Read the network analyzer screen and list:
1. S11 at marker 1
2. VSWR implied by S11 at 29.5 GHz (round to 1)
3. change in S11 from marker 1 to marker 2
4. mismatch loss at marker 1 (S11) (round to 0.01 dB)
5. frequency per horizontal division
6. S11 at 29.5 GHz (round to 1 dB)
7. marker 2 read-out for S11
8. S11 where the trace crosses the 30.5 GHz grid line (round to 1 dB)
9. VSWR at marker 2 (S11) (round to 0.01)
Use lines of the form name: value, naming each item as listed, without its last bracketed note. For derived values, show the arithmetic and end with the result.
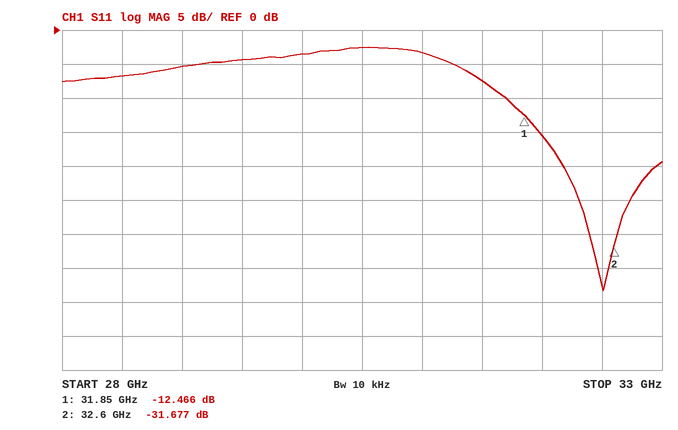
S11 at marker 1: -12.466 dB
VSWR implied by S11 at 29.5 GHz: |Γ| = 10^(-4/20) = 0.6310; VSWR = (1 + 0.6310)/(1 − 0.6310) ≈ 4
change in S11 from marker 1 to marker 2: -31.677 − (-12.466) = -19.211 dB
mismatch loss at marker 1 (S11): −10 log10(1 − 10^(-12.466/10)) ≈ 0.25 dB
frequency per horizontal division: 500 MHz
S11 at 29.5 GHz: -4 dB
marker 2 read-out for S11: -31.677 dB
S11 where the trace crosses the 30.5 GHz grid line: -3 dB
VSWR at marker 2 (S11): (1 + 0.0261)/(1 − 0.0261) ≈ 1.05
